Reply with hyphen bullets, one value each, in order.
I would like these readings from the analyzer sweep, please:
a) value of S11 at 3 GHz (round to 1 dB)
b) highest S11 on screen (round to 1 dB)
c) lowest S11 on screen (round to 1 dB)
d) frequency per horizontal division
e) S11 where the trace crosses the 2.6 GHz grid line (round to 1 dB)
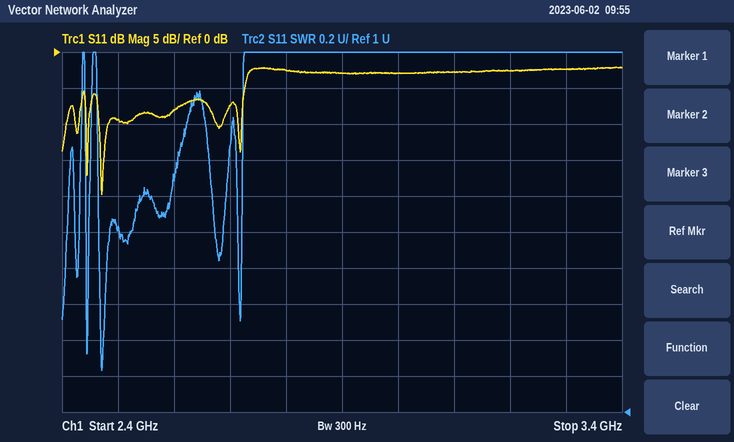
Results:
- -3 dB
- -2 dB
- -20 dB
- 100 MHz
- -8 dB
